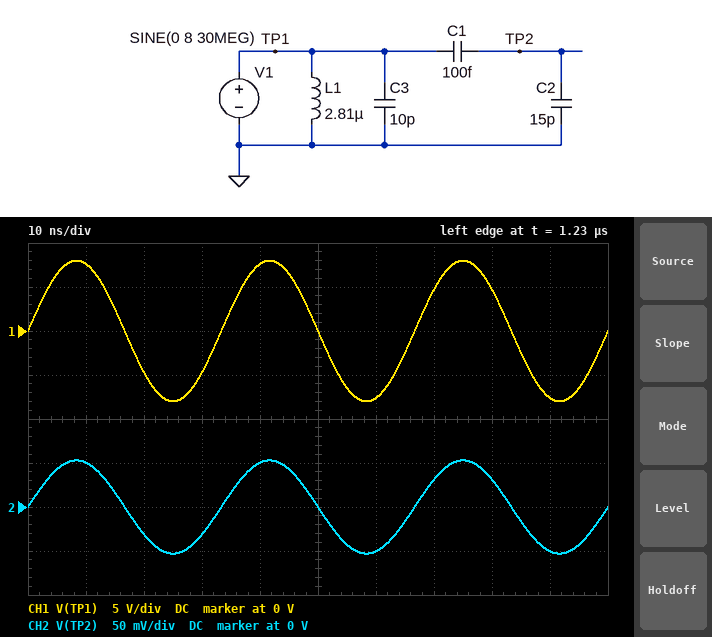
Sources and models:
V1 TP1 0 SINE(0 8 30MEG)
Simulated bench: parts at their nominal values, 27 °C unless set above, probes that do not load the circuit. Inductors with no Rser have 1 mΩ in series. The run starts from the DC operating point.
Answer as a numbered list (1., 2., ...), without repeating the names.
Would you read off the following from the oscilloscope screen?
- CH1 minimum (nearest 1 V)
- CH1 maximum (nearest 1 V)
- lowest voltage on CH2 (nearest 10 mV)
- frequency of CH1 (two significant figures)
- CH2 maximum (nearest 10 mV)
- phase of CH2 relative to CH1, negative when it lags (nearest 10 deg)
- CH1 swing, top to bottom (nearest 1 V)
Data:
1. -8 V
2. 8 V
3. -50 mV
4. 30 MHz
5. 50 mV
6. 0 deg
7. 16 V
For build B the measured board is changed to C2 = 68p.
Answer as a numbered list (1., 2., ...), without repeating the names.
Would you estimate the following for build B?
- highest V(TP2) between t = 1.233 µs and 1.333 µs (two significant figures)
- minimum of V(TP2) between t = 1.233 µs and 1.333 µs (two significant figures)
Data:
1. 12 mV
2. -12 mV
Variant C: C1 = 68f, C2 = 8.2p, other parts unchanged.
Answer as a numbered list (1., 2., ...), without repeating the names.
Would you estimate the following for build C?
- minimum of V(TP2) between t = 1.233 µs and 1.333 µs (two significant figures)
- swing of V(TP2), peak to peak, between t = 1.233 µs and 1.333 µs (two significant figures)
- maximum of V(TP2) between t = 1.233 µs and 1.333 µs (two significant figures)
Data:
1. -66 mV
2. 130 mV
3. 66 mV
